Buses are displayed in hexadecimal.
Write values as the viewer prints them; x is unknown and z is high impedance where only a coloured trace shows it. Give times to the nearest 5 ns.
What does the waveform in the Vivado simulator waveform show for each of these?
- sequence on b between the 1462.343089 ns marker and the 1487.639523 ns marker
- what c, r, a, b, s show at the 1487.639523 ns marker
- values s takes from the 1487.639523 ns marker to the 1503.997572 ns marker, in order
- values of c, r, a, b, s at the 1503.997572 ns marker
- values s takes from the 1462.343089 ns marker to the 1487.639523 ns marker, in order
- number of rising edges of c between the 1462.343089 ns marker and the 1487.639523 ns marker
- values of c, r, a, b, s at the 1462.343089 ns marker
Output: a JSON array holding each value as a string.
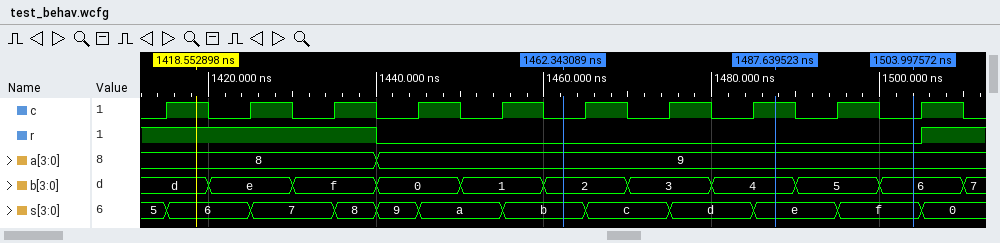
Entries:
["2, 3, 4", "c=1, r=0, a=9, b=4, s=e", "e, f", "c=0, r=0, a=9, b=6, s=f", "b, c, d, e", "3", "c=0, r=0, a=9, b=2, s=b"]
